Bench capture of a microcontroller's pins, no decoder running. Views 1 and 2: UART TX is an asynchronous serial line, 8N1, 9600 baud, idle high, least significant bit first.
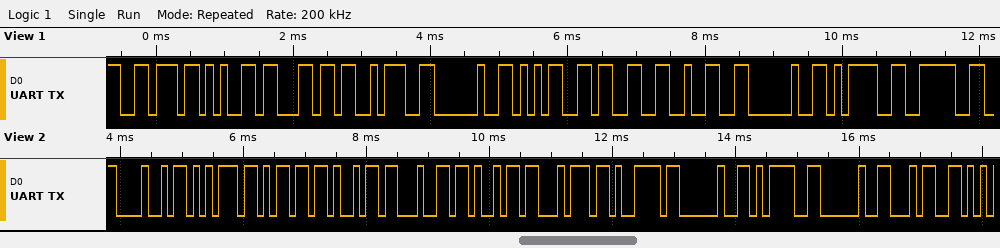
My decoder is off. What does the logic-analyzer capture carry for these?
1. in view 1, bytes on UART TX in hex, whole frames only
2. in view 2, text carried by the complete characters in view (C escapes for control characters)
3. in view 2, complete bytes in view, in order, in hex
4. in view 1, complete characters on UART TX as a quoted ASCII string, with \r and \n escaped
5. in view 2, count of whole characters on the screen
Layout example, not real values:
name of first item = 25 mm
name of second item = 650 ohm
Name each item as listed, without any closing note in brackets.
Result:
in view 1, bytes on UART TX in hex, whole frames only = 76 65 6C 3A 20 35 33 32 20 3D 3E
in view 2, text carried by the complete characters in view = "Humidity = 4"
in view 2, complete bytes in view, in order, in hex = 0x48 0x75 0x6D 0x69 0x64 0x69 0x74 0x79 0x20 0x3D 0x20 0x34
in view 1, complete characters on UART TX as a quoted ASCII string, with \r and \n escaped = "vel: 532 =>"
in view 2, count of whole characters on the screen = 12
